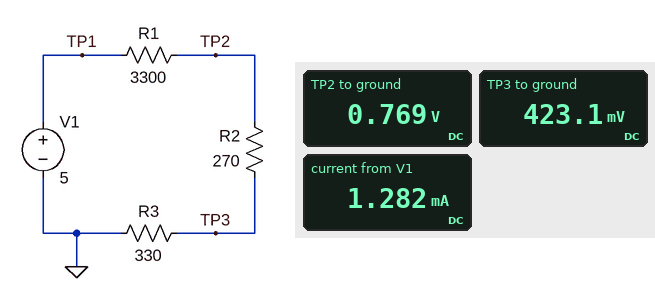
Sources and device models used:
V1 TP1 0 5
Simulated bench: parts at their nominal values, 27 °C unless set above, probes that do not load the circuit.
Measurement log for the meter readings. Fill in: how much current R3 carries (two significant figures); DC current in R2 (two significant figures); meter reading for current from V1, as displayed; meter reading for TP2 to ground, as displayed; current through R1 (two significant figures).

1.3 mA
1.3 mA
1.282 mA
0.769 V
1.3 mA
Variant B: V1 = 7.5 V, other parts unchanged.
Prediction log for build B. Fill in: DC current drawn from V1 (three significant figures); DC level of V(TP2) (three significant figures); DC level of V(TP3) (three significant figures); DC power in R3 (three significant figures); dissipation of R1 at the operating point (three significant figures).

1.92 mA
1.15 V
635 mV
1.22 mW
12.2 mW
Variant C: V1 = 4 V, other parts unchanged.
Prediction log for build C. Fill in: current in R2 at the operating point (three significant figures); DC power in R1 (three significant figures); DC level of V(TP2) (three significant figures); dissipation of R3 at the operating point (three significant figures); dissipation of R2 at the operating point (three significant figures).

1.03 mA
3.47 mW
615 mV
347 µW
284 µW
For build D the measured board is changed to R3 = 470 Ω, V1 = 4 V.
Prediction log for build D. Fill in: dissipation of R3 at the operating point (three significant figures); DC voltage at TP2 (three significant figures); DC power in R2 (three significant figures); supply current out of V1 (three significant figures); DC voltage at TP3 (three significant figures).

461 µW
733 mV
265 µW
990 µA
465 mV
